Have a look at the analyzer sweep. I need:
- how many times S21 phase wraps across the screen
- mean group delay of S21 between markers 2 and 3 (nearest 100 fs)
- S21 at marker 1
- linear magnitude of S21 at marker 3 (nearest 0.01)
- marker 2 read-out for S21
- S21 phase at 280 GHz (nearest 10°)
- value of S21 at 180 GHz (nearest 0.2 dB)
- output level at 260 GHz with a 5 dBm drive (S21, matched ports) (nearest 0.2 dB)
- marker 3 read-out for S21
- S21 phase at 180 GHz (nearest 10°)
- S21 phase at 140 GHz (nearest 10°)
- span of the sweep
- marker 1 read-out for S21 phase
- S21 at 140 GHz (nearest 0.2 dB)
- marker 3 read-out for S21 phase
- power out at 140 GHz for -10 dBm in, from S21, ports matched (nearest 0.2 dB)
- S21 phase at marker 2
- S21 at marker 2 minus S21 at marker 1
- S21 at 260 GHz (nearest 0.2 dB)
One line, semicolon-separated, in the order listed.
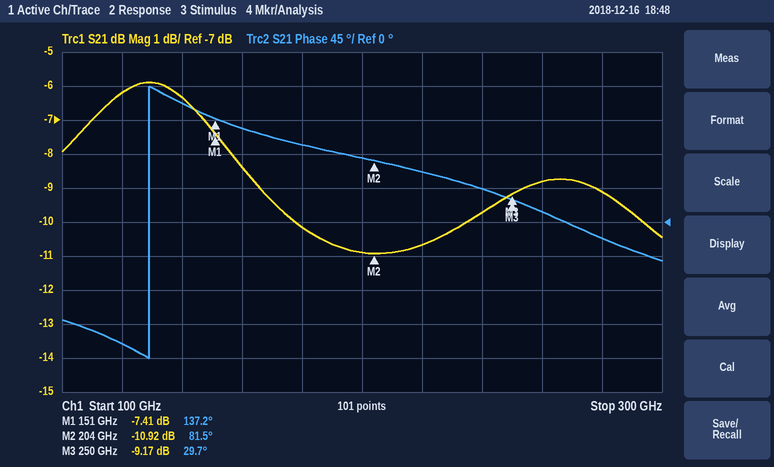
1; 3.1 ps; -7.41 dB; 0.35; -10.92 dB; -20°; -10.2 dB; -3.8 dBm; -9.17 dB; 100°; 160°; 200 GHz; 137.2°; -6.4 dB; 29.7°; -16.4 dBm; 81.5°; -3.51 dB; -8.8 dB
